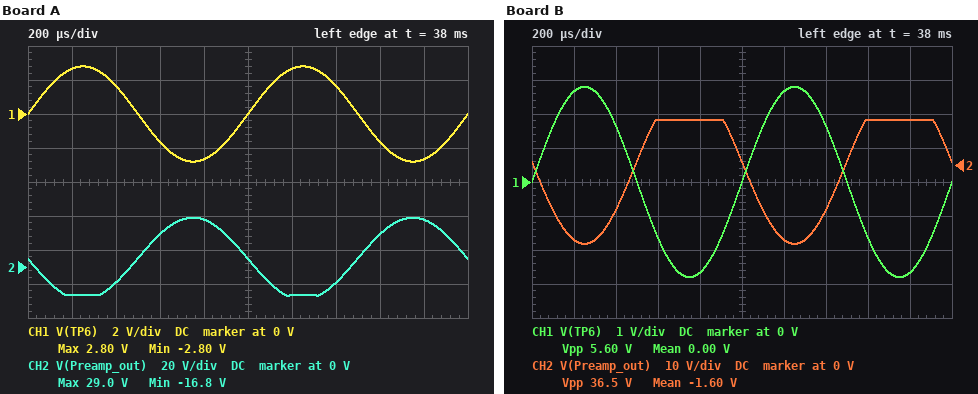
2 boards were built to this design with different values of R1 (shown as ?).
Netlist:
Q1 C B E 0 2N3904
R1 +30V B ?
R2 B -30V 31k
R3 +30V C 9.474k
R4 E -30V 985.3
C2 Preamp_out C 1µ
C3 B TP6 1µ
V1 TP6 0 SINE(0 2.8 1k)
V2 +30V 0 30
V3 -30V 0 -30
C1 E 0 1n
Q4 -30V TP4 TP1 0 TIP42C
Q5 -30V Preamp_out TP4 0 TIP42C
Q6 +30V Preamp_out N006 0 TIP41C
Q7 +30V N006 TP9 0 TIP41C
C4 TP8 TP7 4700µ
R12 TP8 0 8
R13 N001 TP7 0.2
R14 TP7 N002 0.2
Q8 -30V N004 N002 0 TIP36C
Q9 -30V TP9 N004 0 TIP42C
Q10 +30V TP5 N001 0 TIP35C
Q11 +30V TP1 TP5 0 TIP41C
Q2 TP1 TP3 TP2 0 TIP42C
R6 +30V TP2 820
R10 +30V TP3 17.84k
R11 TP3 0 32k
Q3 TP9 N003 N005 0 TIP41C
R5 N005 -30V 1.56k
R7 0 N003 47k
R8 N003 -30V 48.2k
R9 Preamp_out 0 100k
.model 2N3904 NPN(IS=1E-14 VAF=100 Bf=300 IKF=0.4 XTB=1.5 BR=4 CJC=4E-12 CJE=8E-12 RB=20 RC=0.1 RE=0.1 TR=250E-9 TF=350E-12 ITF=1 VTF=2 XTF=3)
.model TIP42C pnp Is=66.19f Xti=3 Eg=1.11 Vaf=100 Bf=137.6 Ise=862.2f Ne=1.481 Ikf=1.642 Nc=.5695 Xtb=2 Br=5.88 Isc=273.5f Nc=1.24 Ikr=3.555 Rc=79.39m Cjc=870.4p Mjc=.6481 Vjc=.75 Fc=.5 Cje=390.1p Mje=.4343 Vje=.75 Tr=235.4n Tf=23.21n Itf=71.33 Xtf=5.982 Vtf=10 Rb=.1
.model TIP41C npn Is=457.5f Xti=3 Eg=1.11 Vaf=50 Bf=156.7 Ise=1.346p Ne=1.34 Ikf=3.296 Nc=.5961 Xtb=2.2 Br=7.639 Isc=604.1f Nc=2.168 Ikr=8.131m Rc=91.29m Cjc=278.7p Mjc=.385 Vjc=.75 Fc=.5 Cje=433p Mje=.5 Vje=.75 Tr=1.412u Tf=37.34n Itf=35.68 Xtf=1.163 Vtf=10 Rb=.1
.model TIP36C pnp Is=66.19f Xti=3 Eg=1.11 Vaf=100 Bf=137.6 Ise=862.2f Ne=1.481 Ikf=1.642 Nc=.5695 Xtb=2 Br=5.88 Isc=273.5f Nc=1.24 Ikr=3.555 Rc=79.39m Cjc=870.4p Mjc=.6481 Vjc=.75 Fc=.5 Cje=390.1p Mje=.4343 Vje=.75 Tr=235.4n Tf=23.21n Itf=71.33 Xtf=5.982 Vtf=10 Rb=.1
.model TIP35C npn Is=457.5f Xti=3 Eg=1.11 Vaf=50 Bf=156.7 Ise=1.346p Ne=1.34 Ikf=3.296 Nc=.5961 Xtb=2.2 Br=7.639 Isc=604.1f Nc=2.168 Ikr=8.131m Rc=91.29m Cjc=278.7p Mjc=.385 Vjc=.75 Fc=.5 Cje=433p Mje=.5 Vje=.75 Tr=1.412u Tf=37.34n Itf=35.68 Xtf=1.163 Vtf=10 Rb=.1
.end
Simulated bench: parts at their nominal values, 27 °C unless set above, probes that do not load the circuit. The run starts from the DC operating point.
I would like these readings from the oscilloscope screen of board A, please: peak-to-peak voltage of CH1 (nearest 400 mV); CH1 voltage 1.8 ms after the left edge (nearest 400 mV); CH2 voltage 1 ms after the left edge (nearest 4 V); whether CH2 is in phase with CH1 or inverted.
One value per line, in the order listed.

5.6 V
-2.8 V
4 V
inverted
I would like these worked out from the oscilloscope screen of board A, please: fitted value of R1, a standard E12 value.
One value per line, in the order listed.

330 kΩ
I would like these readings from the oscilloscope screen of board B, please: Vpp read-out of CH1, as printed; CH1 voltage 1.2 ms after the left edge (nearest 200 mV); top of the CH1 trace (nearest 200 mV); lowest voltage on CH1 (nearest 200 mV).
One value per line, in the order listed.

5.60 V
2.6 V
2.8 V
-2.8 V
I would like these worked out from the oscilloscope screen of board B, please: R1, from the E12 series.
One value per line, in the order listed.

820 kΩ
